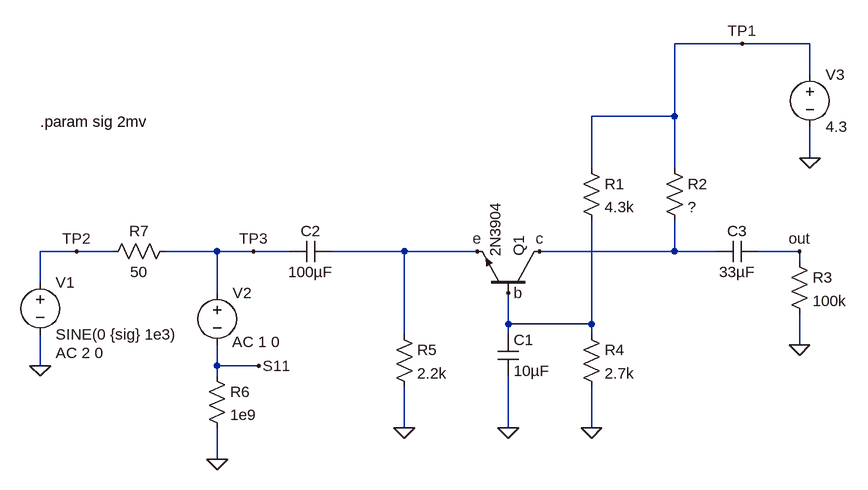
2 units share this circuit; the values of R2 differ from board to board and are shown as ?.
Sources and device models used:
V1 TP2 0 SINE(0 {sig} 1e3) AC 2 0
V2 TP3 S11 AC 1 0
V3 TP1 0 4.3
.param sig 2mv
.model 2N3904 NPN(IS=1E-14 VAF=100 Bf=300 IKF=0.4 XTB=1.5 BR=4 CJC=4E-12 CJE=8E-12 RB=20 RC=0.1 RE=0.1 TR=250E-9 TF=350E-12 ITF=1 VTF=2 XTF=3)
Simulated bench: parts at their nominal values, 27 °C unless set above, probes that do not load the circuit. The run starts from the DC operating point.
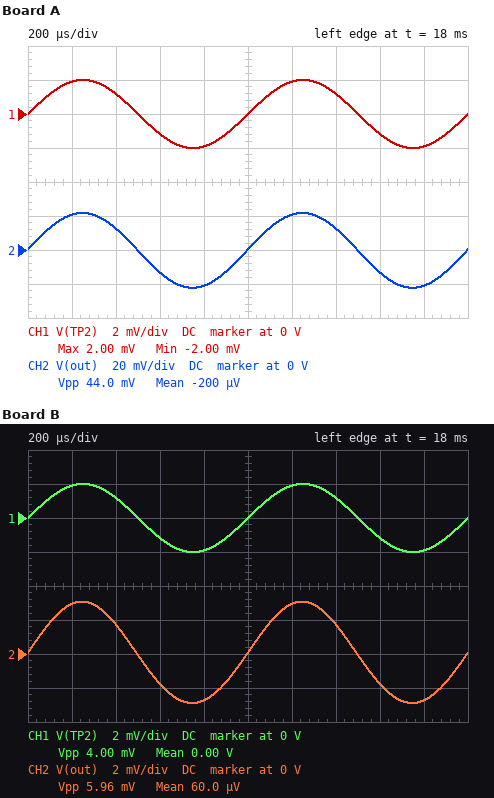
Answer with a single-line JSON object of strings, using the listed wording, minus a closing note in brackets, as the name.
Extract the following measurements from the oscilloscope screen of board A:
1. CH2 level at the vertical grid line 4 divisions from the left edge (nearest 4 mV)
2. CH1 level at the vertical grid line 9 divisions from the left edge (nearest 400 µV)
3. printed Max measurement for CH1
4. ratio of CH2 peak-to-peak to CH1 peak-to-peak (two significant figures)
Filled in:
{"CH2 level at the vertical grid line 4 divisions from the left edge": "-20 mV", "CH1 level at the vertical grid line 9 divisions from the left edge": "-2.0 mV", "printed Max measurement for CH1": "2.00 mV", "ratio of CH2 peak-to-peak to CH1 peak-to-peak": "11"}
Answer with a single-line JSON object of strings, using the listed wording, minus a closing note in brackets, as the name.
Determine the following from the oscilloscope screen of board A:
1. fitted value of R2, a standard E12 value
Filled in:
{"fitted value of R2, a standard E12 value": "1.2 kΩ"}
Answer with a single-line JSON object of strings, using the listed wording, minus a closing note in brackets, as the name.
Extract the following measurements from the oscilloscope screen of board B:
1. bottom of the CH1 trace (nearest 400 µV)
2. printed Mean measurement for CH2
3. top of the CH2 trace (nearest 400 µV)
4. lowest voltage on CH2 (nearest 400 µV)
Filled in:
{"bottom of the CH1 trace": "-2.0 mV", "printed Mean measurement for CH2": "60.0 µV", "top of the CH2 trace": "3.2 mV", "lowest voltage on CH2": "-2.8 mV"}
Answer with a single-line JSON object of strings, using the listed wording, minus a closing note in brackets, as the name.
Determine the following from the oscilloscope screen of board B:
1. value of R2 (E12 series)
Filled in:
{"value of R2": "10 kΩ"}
